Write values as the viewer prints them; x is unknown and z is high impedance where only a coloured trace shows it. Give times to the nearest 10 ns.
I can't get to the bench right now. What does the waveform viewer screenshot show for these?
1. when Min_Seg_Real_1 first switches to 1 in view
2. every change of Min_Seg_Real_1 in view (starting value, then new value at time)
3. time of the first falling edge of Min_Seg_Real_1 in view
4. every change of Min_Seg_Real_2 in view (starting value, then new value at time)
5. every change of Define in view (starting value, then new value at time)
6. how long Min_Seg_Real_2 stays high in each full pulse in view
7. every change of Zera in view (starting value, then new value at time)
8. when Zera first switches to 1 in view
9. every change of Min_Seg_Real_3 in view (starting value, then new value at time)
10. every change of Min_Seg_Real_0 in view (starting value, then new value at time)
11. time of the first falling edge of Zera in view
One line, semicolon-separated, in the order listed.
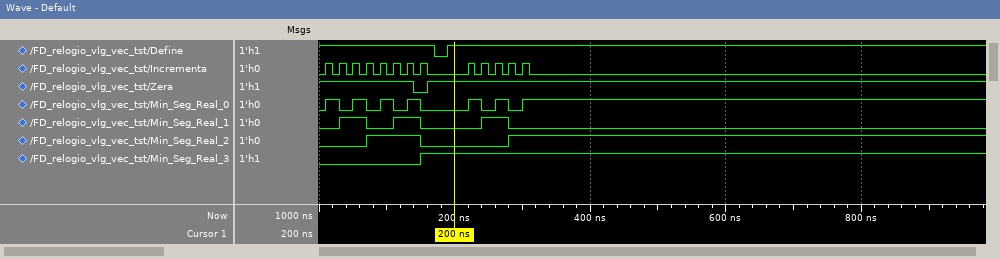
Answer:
30 ns; 0, 1 at 30 ns, 0 at 70 ns, 1 at 110 ns, 0 at 150 ns, 1 at 240 ns, 0 at 280 ns; 70 ns; 0, 1 at 70 ns, 0 at 150 ns, 1 at 280 ns; 1, 0 at 170 ns, 1 at 190 ns; 80 ns; 1, 0 at 140 ns, 1 at 160 ns; 160 ns; 0, 1 at 150 ns; 0, 1 at 10 ns, 0 at 30 ns, 1 at 50 ns, 0 at 70 ns, 1 at 90 ns, 0 at 110 ns, 1 at 130 ns, 0 at 150 ns, 1 at 220 ns, 0 at 240 ns, 1 at 260 ns, 0 at 280 ns, 1 at 300 ns; 140 ns
